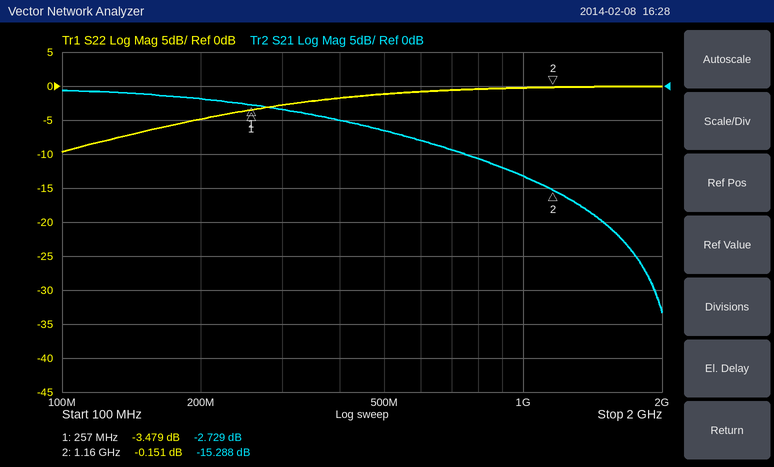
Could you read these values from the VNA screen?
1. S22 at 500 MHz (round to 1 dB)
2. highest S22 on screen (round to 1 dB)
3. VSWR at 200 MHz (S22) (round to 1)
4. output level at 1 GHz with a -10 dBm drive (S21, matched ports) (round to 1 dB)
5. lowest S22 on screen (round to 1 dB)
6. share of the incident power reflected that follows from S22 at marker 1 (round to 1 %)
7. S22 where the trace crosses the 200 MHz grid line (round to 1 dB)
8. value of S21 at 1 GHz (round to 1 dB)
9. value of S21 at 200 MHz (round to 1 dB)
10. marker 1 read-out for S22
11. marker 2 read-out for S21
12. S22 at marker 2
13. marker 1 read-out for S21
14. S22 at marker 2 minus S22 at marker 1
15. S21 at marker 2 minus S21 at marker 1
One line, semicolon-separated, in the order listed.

-1 dB; 0 dB; 4; -23 dBm; -10 dB; 45 %; -5 dB; -13 dB; -2 dB; -3.479 dB; -15.288 dB; -0.151 dB; -2.729 dB; 3.328 dB; -12.559 dB
